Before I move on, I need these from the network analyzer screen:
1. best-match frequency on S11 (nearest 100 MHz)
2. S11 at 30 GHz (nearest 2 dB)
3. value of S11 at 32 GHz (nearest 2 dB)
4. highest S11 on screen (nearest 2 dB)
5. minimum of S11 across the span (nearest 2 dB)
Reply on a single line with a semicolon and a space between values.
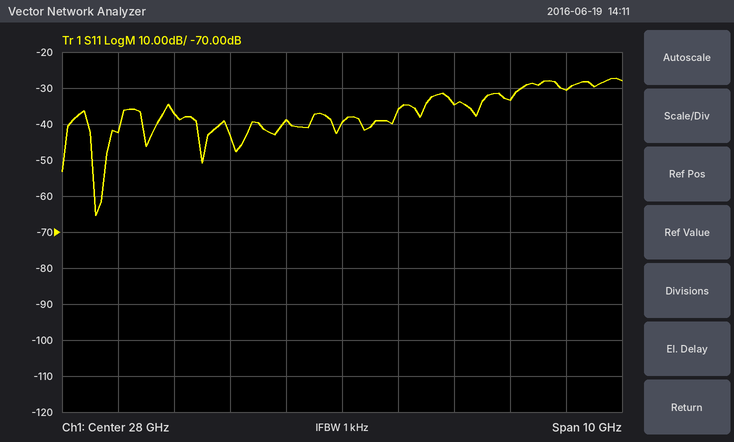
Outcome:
23.6 GHz; -34 dB; -30 dB; -28 dB; -66 dB
